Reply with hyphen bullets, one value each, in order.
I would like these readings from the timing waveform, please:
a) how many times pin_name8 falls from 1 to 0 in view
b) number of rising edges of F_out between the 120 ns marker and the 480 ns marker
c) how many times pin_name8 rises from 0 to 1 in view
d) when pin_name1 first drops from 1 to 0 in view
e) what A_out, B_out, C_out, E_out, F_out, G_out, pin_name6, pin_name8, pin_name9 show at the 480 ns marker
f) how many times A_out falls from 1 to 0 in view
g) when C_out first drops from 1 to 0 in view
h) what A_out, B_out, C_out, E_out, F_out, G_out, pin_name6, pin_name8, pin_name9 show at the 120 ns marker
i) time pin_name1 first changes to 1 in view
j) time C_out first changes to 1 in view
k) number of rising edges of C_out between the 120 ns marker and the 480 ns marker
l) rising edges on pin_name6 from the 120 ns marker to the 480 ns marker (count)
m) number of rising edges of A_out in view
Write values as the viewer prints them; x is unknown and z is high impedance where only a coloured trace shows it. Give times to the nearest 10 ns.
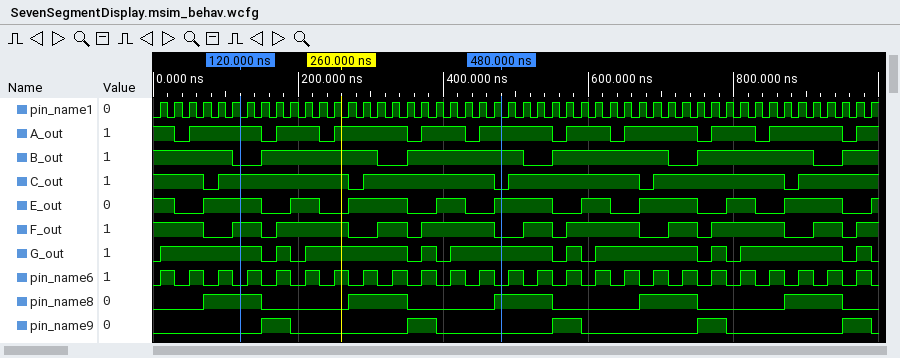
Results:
- 5
- 3
- 5
- 20 ns
- A_out=1, B_out=1, C_out=0, E_out=1, F_out=0, G_out=1, pin_name6=0, pin_name8=1, pin_name9=0
- 10
- 70 ns
- A_out=1, B_out=0, C_out=1, E_out=1, F_out=1, G_out=1, pin_name6=0, pin_name8=1, pin_name9=0
- 10 ns
- 90 ns
- 1
- 9
- 10
